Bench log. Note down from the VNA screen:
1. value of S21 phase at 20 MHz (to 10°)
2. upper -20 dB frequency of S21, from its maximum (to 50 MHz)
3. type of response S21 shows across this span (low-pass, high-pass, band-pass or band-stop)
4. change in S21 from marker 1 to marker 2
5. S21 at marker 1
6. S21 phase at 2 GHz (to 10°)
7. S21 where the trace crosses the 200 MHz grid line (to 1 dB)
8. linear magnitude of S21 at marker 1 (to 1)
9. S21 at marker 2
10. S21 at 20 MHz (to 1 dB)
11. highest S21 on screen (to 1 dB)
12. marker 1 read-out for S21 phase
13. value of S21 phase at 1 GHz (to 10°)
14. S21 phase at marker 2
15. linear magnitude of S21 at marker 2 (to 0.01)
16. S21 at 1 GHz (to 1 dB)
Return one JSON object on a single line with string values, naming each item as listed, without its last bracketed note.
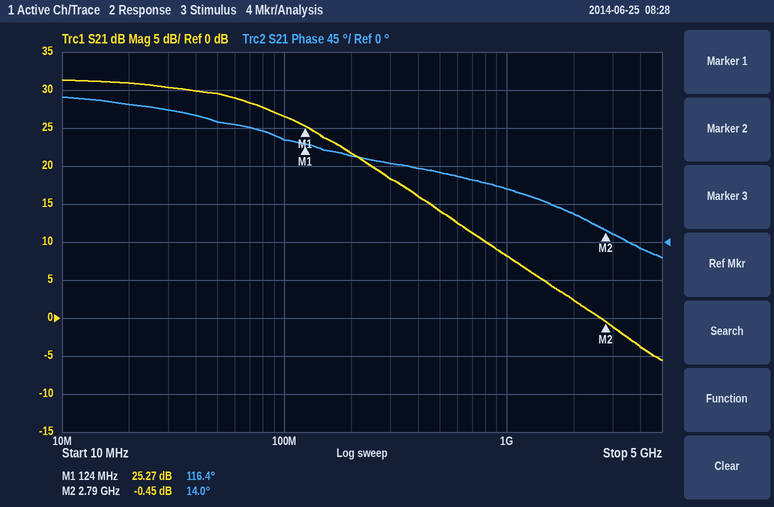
{"value of S21 phase at 20 MHz": "160°", "upper -20 dB frequency of S21, from its maximum": "700 MHz", "type of response S21 shows across this span": "low-pass", "change in S21 from marker 1 to marker 2": "-25.72 dB", "S21 at marker 1": "25.27 dB", "S21 phase at 2 GHz": "30°", "S21 where the trace crosses the 200 MHz grid line": "22 dB", "linear magnitude of S21 at marker 1": "18", "S21 at marker 2": "-0.45 dB", "S21 at 20 MHz": "31 dB", "highest S21 on screen": "31 dB", "marker 1 read-out for S21 phase": "116.4°", "value of S21 phase at 1 GHz": "60°", "S21 phase at marker 2": "14.0°", "linear magnitude of S21 at marker 2": "0.95", "S21 at 1 GHz": "8 dB"}
